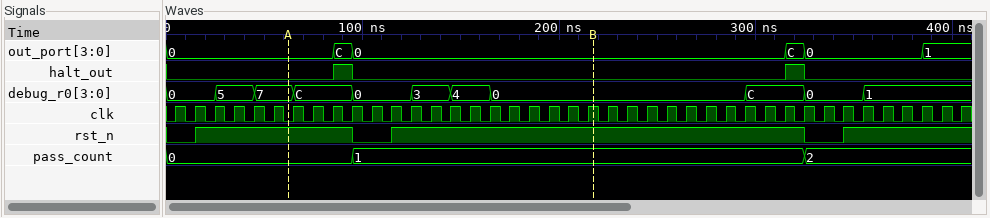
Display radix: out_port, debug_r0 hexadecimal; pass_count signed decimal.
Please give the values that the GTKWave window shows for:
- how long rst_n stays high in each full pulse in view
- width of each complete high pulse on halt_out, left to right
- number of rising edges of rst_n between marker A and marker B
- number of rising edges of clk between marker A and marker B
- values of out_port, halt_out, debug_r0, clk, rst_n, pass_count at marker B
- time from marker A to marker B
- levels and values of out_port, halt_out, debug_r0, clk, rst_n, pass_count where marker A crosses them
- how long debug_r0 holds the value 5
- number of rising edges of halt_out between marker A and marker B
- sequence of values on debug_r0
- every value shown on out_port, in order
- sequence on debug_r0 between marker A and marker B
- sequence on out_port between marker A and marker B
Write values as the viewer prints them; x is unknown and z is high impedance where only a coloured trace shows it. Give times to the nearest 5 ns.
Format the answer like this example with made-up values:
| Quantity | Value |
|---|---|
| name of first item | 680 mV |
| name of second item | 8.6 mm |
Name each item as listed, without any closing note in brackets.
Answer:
| Quantity | Value |
|---|---|
| how long rst_n stays high in each full pulse in view | 80 ns, 210 ns |
| width of each complete high pulse on halt_out, left to right | 10 ns, 10 ns |
| number of rising edges of rst_n between marker A and marker B | 1 |
| number of rising edges of clk between marker A and marker B | 16 |
| values of out_port, halt_out, debug_r0, clk, rst_n, pass_count at marker B | out_port=0, halt_out=0, debug_r0=0, clk=1, rst_n=1, pass_count=1 |
| time from marker A to marker B | 155 ns |
| levels and values of out_port, halt_out, debug_r0, clk, rst_n, pass_count where marker A crosses them | out_port=0, halt_out=0, debug_r0=7, clk=0, rst_n=1, pass_count=0 |
| how long debug_r0 holds the value 5 | 20 ns |
| number of rising edges of halt_out between marker A and marker B | 1 |
| sequence of values on debug_r0 | 0, 5, 7, C, 0, 3, 4, 0, C, 0, 1 |
| every value shown on out_port, in order | 0, C, 0, C, 0, 1 |
| sequence on debug_r0 between marker A and marker B | 7, C, 0, 3, 4, 0 |
| sequence on out_port between marker A and marker B | 0, C, 0 |
